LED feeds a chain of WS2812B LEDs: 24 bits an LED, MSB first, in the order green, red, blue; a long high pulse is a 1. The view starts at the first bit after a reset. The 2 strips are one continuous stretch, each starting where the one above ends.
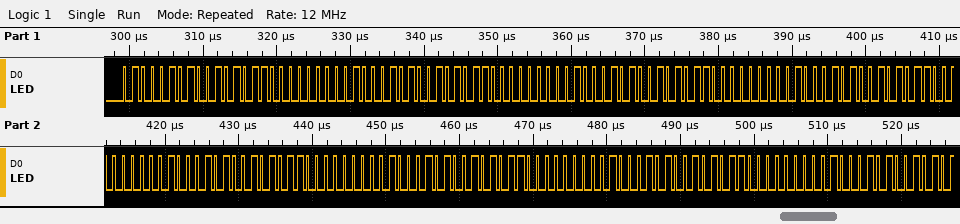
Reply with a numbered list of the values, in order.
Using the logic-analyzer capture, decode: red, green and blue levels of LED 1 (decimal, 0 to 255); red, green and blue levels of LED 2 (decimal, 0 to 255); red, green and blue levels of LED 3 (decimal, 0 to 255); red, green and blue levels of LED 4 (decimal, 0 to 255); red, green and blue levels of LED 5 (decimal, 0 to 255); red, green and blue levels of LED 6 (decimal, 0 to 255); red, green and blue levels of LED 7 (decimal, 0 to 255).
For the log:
1. 43, 69, 0
2. 43, 69, 0
3. 43, 69, 0
4. 43, 69, 0
5. 43, 69, 0
6. 43, 69, 0
7. 43, 69, 0
